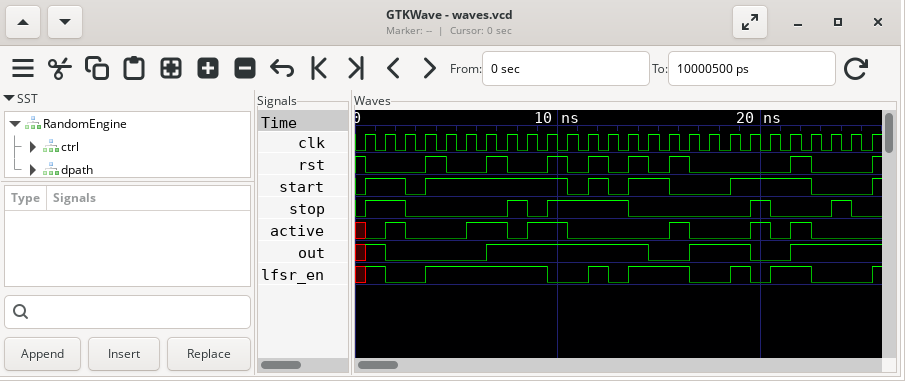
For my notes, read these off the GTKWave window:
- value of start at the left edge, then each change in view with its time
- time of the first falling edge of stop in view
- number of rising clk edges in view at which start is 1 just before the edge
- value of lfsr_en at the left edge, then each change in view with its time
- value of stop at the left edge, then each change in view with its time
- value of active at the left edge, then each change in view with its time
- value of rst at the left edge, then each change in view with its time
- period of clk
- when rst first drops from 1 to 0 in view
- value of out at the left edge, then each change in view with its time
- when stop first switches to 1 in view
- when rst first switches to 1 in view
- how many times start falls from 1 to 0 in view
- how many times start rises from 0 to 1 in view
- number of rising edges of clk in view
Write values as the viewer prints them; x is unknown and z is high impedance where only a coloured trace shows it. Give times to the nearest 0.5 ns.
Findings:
0, 1 at 0.5 ns, 0 at 2.5 ns, 1 at 3.5 ns, 0 at 10.5 ns, 1 at 11.5 ns, 0 at 12.5 ns, 1 at 13.5 ns, 0 at 15.5 ns, 1 at 18.5 ns, 0 at 22.5 ns, 1 at 25.5 ns
2.5 ns
16
x, 1 at 0.5 ns, 0 at 1.5 ns, 1 at 3.5 ns, 0 at 9.5 ns, 1 at 11.5 ns, 0 at 12.5 ns, 1 at 13.5 ns, 0 at 16.5 ns, 1 at 18.5 ns, 0 at 19.5 ns, 1 at 20.5 ns, 0 at 22.5 ns, 1 at 25.5 ns
0, 1 at 0.5 ns, 0 at 2.5 ns, 1 at 7.5 ns, 0 at 8.5 ns, 1 at 9.5 ns, 0 at 13.5 ns, 1 at 19.5 ns, 0 at 20.5 ns, 1 at 23.5 ns, 0 at 24.5 ns
x, 0 at 0.5 ns, 1 at 1.5 ns, 0 at 2.5 ns, 1 at 5.5 ns, 0 at 7.5 ns, 1 at 8.5 ns, 0 at 10.5 ns, 1 at 15.5 ns, 0 at 16.5 ns, 1 at 19.5 ns, 0 at 20.5 ns, 1 at 21.5 ns, 0 at 22.5 ns
1, 0 at 0.5 ns, 1 at 3.5 ns, 0 at 4.5 ns, 1 at 6.5 ns, 0 at 7.5 ns, 1 at 9.5 ns, 0 at 10.5 ns, 1 at 11.5 ns, 0 at 12.5 ns, 1 at 13.5 ns, 0 at 14.5 ns, 1 at 15.5 ns, 0 at 16.5 ns, 1 at 21.5 ns, 0 at 22.5 ns, 1 at 25.5 ns
1 ns
0.5 ns
x, 1 at 0.5 ns, 0 at 1.5 ns, 1 at 6.5 ns, 0 at 14.5 ns, 1 at 16.5 ns, 0 at 19.5 ns, 1 at 21.5 ns
0.5 ns
3.5 ns
5
6
26
